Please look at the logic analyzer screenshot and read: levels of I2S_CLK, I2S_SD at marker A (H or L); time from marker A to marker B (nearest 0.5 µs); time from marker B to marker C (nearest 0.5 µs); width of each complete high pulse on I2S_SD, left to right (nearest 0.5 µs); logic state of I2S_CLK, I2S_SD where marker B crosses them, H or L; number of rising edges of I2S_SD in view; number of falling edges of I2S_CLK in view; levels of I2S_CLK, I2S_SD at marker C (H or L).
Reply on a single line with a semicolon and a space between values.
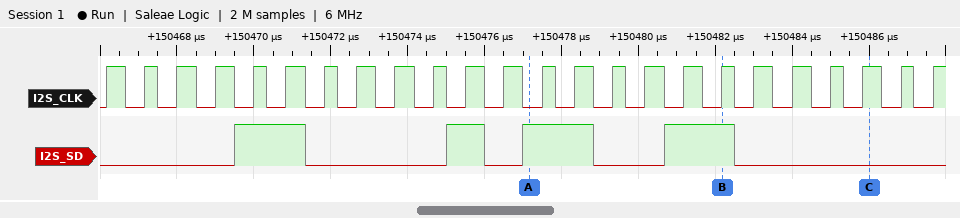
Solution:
I2S_CLK=L, I2S_SD=H; 5 µs; 4 µs; 2 µs, 1 µs, 2 µs, 2 µs; I2S_CLK=H, I2S_SD=H; 4; 23; I2S_CLK=H, I2S_SD=L
